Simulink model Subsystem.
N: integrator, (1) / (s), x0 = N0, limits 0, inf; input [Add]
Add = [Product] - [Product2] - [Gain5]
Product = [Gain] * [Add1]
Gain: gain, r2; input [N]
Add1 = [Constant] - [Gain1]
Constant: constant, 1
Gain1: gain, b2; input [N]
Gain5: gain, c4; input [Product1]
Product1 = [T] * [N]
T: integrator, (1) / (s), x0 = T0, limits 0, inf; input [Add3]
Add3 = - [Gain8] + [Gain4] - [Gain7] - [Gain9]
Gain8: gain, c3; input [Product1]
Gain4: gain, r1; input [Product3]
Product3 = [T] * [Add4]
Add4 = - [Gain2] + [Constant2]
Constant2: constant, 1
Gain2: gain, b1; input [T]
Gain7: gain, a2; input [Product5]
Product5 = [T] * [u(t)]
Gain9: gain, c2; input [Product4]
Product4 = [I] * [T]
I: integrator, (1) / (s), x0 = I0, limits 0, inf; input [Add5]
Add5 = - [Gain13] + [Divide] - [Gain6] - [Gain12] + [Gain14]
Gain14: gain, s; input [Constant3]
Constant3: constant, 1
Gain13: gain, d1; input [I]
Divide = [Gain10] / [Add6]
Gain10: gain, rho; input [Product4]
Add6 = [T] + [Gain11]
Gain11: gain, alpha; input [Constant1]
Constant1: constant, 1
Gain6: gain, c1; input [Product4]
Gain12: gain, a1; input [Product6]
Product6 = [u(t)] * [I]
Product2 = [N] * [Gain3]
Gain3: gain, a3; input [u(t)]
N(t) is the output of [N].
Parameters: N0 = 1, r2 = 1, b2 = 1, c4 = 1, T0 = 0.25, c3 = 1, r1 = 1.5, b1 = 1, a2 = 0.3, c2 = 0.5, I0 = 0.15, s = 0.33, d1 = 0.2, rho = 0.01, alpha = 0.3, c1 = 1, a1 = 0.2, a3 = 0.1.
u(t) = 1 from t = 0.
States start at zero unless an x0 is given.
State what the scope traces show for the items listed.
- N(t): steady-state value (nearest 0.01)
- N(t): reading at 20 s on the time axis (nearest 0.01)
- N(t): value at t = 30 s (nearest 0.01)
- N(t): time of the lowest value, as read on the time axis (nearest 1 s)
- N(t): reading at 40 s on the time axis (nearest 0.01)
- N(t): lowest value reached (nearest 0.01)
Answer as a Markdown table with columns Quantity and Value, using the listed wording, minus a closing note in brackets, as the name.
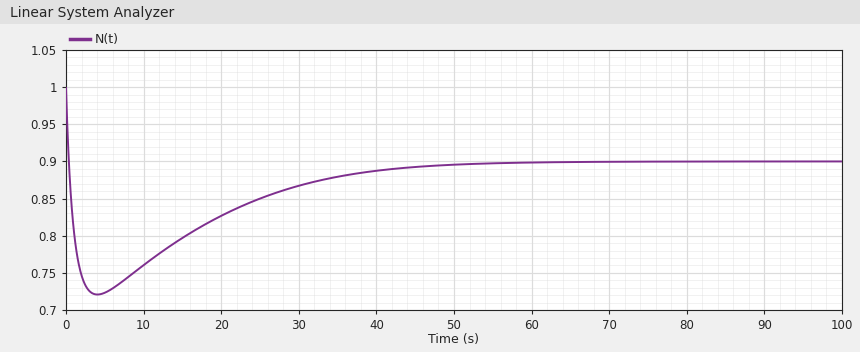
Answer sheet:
| Quantity | Value |
|---|---|
| N(t): steady-state value | 0.90 |
| N(t): reading at 20 s on the time axis | 0.83 |
| N(t): value at t = 30 s | 0.87 |
| N(t): time of the lowest value, as read on the time axis | 4 s |
| N(t): reading at 40 s on the time axis | 0.89 |
| N(t): lowest value reached | 0.72 |
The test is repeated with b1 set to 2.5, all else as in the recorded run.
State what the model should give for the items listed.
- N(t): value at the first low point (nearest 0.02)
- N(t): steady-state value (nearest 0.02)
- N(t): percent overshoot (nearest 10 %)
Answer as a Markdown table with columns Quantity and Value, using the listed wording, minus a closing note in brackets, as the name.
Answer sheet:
| Quantity | Value |
|---|---|
| N(t): value at the first low point | 0.80 |
| N(t): steady-state value | 0.90 |
| N(t): percent overshoot | 100 % |
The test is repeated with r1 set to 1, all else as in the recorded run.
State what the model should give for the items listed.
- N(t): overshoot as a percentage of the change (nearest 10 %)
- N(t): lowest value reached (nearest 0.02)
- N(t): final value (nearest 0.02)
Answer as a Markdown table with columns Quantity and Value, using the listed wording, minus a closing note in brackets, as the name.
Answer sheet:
| Quantity | Value |
|---|---|
| N(t): overshoot as a percentage of the change | 100 % |
| N(t): lowest value reached | 0.80 |
| N(t): final value | 0.90 |
